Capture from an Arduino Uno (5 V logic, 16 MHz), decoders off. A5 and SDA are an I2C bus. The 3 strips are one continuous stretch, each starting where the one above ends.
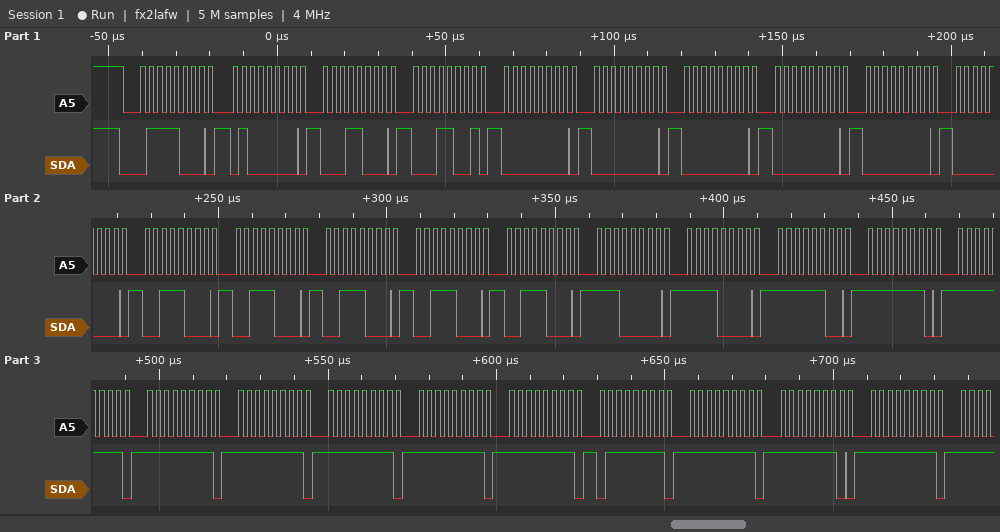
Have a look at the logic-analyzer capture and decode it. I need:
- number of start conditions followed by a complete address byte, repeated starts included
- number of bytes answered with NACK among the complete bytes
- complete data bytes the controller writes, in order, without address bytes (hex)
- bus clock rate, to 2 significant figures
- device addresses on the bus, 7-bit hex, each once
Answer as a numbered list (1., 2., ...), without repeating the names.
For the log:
1. 1
2. 0
3. 40 18 19 00 00 00 00 00 00 38 38 38 38 38 E0 F0 FC FE FF FF FF FF FF FF 7F FF FE FF
4. 400 kHz
5. 0x3C
